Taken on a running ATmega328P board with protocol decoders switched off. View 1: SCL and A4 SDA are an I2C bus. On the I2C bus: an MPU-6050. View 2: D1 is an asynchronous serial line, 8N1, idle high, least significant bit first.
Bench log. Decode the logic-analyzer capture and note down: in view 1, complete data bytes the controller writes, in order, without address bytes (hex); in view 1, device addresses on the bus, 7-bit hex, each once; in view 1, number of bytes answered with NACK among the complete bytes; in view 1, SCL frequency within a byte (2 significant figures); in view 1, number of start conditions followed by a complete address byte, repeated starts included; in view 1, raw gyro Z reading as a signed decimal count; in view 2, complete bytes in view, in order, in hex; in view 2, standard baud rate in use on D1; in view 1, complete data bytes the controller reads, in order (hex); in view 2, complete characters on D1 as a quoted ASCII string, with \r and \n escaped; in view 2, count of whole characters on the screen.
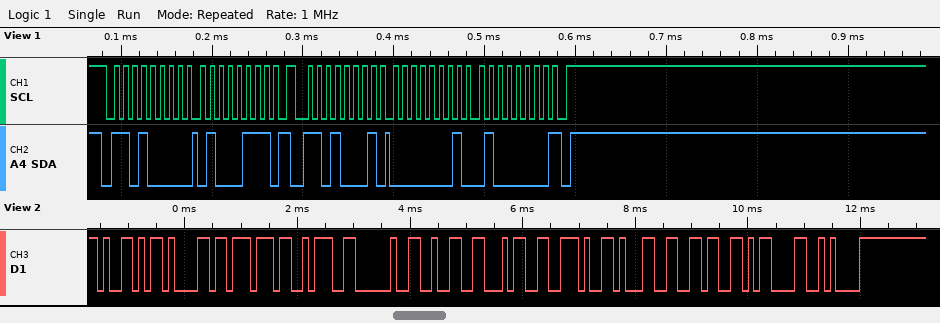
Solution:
47
0x68
1
100 kHz
2
320
0x59 0x61 0x77 0x3A 0x20 0x32 0x34 0x2E 0x31 0x36 0x0D 0x0A
9600 baud
01 40
"Yaw: 24.16\r\n"
12
